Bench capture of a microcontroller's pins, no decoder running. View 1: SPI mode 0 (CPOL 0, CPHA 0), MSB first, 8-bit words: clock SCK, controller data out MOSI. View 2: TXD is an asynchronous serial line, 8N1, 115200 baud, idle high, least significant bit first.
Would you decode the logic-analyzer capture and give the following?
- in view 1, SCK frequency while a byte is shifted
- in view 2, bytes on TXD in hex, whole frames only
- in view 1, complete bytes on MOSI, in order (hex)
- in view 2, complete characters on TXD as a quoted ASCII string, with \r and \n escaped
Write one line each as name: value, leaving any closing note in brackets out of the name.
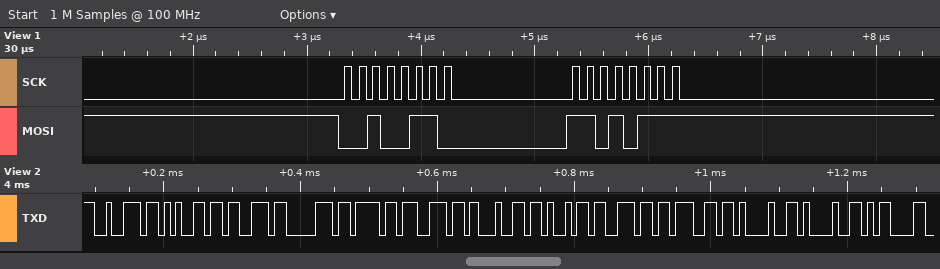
in view 1, SCK frequency while a byte is shifted: 8 MHz
in view 2, bytes on TXD in hex, whole frames only: 72 65 73 70 6F 6E 64 69 6E 67 21 21 0D
in view 1, complete bytes on MOSI, in order: 26 D7
in view 2, complete characters on TXD as a quoted ASCII string, with \r and \n escaped: "responding!!\r"
